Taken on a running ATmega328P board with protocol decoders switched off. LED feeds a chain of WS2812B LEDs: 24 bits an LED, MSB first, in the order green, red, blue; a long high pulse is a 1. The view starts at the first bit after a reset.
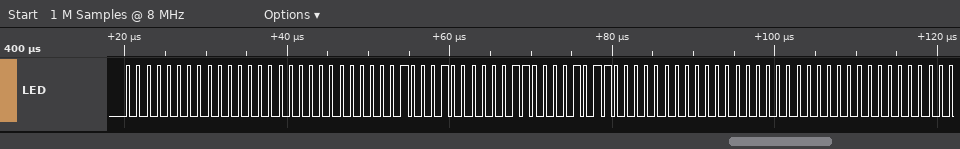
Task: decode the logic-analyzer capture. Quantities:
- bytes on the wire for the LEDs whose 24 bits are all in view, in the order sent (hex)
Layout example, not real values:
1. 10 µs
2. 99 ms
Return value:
1. 00 00 00 11 03 0B 00 00 00
